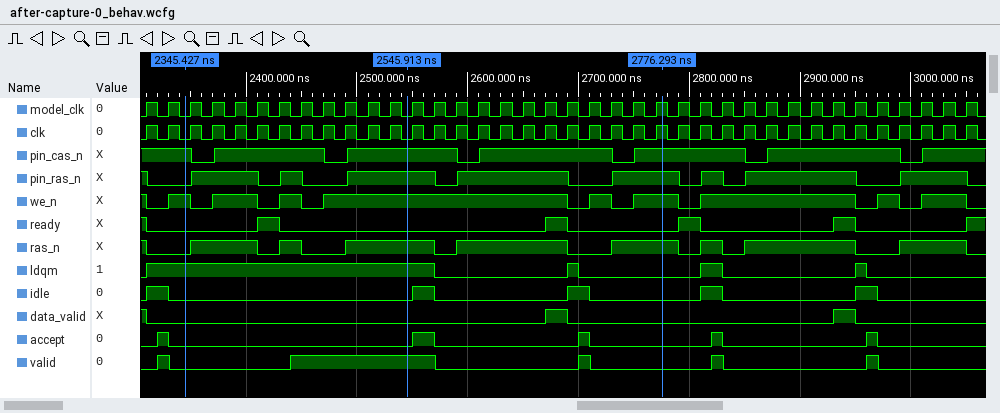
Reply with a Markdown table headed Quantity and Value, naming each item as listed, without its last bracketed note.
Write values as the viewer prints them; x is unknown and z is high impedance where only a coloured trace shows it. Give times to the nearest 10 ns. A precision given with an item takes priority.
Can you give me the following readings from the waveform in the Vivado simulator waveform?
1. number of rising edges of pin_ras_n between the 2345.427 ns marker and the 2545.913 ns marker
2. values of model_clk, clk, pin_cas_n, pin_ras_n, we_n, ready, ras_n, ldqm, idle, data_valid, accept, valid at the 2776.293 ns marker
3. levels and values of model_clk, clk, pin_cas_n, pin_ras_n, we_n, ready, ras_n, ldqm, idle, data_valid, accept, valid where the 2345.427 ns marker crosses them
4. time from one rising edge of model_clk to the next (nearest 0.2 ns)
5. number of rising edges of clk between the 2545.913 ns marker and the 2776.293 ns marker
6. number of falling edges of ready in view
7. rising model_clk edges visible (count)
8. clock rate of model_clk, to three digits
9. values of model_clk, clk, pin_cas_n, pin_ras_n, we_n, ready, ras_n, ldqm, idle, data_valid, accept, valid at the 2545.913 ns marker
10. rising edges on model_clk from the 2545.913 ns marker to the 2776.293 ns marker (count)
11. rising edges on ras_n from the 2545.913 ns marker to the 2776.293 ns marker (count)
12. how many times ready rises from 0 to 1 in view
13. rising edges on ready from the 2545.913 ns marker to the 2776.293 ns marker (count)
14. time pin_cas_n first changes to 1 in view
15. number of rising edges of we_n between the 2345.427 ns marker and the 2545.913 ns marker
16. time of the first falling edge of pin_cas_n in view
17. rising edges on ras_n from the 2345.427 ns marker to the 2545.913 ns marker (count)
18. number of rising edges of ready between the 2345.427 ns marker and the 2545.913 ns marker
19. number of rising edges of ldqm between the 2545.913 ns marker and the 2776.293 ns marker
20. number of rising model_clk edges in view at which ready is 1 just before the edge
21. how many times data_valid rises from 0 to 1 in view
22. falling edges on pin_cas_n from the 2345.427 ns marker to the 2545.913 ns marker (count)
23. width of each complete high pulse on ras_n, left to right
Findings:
| Quantity | Value |
|---|---|
| number of rising edges of pin_ras_n between the 2345.427 ns marker and the 2545.913 ns marker | 3 |
| values of model_clk, clk, pin_cas_n, pin_ras_n, we_n, ready, ras_n, ldqm, idle, data_valid, accept, valid at the 2776.293 ns marker | model_clk=1, clk=1, pin_cas_n=1, pin_ras_n=1, we_n=1, ready=0, ras_n=1, ldqm=0, idle=0, data_valid=0, accept=0, valid=0 |
| levels and values of model_clk, clk, pin_cas_n, pin_ras_n, we_n, ready, ras_n, ldqm, idle, data_valid, accept, valid where the 2345.427 ns marker crosses them | model_clk=0, clk=0, pin_cas_n=1, pin_ras_n=0, we_n=1, ready=0, ras_n=0, ldqm=1, idle=0, data_valid=0, accept=0, valid=0 |
| time from one rising edge of model_clk to the next | 20 ns |
| number of rising edges of clk between the 2545.913 ns marker and the 2776.293 ns marker | 12 |
| number of falling edges of ready in view | 5 |
| rising model_clk edges visible | 38 |
| clock rate of model_clk, to three digits | 50.0 MHz |
| values of model_clk, clk, pin_cas_n, pin_ras_n, we_n, ready, ras_n, ldqm, idle, data_valid, accept, valid at the 2545.913 ns marker | model_clk=0, clk=0, pin_cas_n=1, pin_ras_n=1, we_n=1, ready=0, ras_n=1, ldqm=1, idle=0, data_valid=0, accept=0, valid=1 |
| rising edges on model_clk from the 2545.913 ns marker to the 2776.293 ns marker | 12 |
| rising edges on ras_n from the 2545.913 ns marker to the 2776.293 ns marker | 2 |
| how many times ready rises from 0 to 1 in view | 5 |
| rising edges on ready from the 2545.913 ns marker to the 2776.293 ns marker | 1 |
| time pin_cas_n first changes to 1 in view | 2370 ns |
| number of rising edges of we_n between the 2345.427 ns marker and the 2545.913 ns marker | 3 |
| time of the first falling edge of pin_cas_n in view | 2350 ns |
| rising edges on ras_n from the 2345.427 ns marker to the 2545.913 ns marker | 3 |
| number of rising edges of ready between the 2345.427 ns marker and the 2545.913 ns marker | 1 |
| number of rising edges of ldqm between the 2545.913 ns marker and the 2776.293 ns marker | 1 |
| number of rising model_clk edges in view at which ready is 1 just before the edge | 5 |
| how many times data_valid rises from 0 to 1 in view | 2 |
| falling edges on pin_cas_n from the 2345.427 ns marker to the 2545.913 ns marker | 2 |
| width of each complete high pulse on ras_n, left to right | 60 ns, 20 ns, 80 ns, 100 ns, 60 ns, 20 ns, 100 ns, 60 ns |
